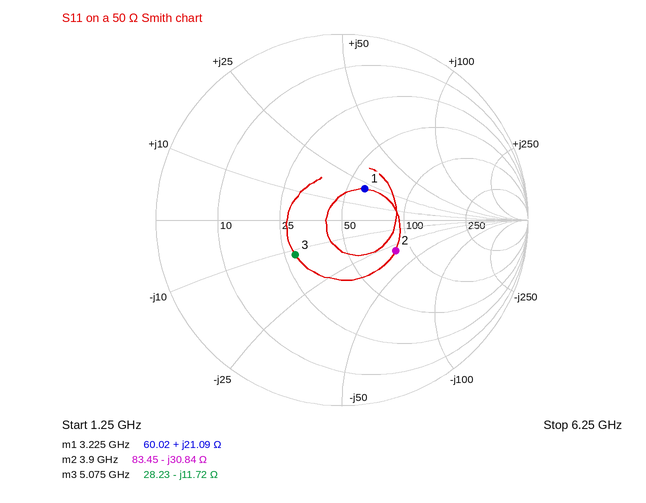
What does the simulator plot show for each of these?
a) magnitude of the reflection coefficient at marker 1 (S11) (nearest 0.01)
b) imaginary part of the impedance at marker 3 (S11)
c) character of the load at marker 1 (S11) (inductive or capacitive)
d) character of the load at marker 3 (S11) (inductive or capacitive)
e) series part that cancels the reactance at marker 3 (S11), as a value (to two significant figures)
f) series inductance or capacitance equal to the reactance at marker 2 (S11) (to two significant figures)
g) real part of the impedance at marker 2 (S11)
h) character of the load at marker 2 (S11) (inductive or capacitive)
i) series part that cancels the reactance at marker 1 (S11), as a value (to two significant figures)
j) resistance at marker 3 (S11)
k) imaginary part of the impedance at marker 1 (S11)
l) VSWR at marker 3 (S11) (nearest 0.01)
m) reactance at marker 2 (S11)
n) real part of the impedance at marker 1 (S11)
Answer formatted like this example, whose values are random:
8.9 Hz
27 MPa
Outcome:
0.21
-11.72 Ω
inductive
capacitive
370 pH
1.3 pF
83.45 Ω
capacitive
2.3 pF
28.23 Ω
+21.09 Ω
1.91
-30.84 Ω
60.02 Ω
